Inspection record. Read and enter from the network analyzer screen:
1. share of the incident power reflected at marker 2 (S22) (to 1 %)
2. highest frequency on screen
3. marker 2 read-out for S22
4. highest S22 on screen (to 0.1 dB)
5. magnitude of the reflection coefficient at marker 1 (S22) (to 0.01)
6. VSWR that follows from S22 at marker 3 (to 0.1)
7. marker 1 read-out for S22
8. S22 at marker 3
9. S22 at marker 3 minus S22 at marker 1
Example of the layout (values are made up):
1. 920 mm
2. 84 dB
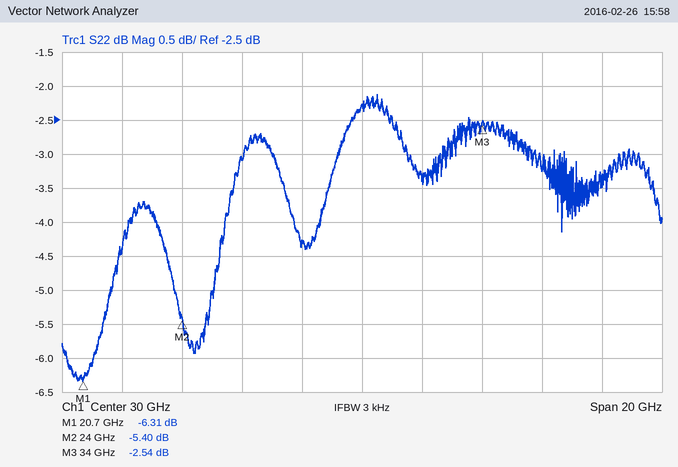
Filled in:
1. 29 %
2. 40 GHz
3. -5.40 dB
4. -2.1 dB
5. 0.48
6. 6.9
7. -6.31 dB
8. -2.54 dB
9. 3.77 dB
